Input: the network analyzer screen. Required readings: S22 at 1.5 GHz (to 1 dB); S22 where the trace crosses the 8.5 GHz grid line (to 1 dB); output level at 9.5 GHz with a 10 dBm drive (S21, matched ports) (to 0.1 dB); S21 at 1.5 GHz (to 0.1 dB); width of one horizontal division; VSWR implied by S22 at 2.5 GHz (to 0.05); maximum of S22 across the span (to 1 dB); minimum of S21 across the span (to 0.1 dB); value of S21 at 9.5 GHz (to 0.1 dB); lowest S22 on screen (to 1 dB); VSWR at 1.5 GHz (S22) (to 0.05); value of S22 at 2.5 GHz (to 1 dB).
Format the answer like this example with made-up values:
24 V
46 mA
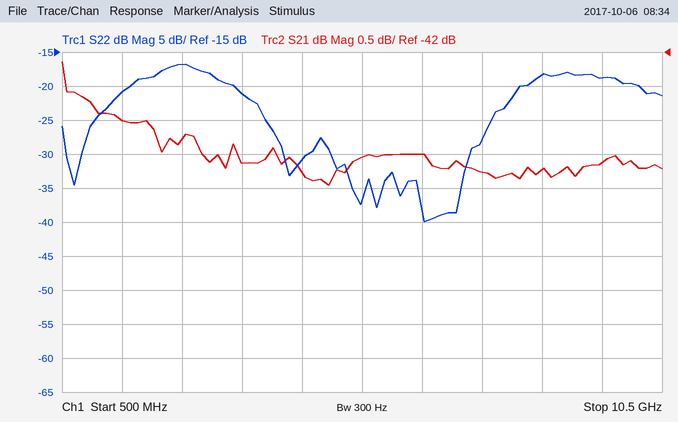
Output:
-21 dB
-18 dB
-33.6 dBm
-43.0 dB
1 GHz
1.35
-17 dB
-44.0 dB
-43.6 dB
-40 dB
1.20
-17 dB
